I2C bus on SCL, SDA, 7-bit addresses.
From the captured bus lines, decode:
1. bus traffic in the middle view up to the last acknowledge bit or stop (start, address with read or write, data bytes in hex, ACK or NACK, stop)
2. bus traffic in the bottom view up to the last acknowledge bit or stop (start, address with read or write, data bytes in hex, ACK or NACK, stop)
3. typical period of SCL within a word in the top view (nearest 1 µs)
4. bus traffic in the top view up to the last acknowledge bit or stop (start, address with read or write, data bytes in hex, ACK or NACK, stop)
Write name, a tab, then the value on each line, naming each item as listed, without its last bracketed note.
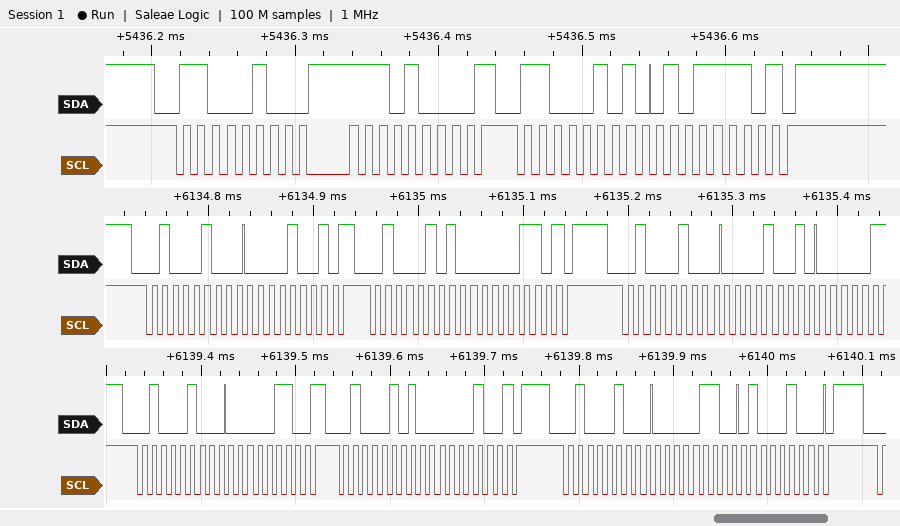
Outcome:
bus traffic in the middle view up to the last acknowledge bit or stop	start, address 22 write ACK, 09 ACK, repeated start, address 22 read ACK, 06 NACK, stop, start, address 22 write ACK, 09 ACK
bus traffic in the bottom view up to the last acknowledge bit or stop	start, address 22 write ACK, 06 ACK, repeated start, address 22 read ACK, 04 NACK, stop, start, address 22 write ACK, 06 ACK, 44 ACK, stop
typical period of SCL within a word in the top view	10 µs
bus traffic in the top view up to the last acknowledge bit or stop	start, address 62 write ACK, E8 ACK, repeated start, address 62 read ACK, 5E NACK, stop
